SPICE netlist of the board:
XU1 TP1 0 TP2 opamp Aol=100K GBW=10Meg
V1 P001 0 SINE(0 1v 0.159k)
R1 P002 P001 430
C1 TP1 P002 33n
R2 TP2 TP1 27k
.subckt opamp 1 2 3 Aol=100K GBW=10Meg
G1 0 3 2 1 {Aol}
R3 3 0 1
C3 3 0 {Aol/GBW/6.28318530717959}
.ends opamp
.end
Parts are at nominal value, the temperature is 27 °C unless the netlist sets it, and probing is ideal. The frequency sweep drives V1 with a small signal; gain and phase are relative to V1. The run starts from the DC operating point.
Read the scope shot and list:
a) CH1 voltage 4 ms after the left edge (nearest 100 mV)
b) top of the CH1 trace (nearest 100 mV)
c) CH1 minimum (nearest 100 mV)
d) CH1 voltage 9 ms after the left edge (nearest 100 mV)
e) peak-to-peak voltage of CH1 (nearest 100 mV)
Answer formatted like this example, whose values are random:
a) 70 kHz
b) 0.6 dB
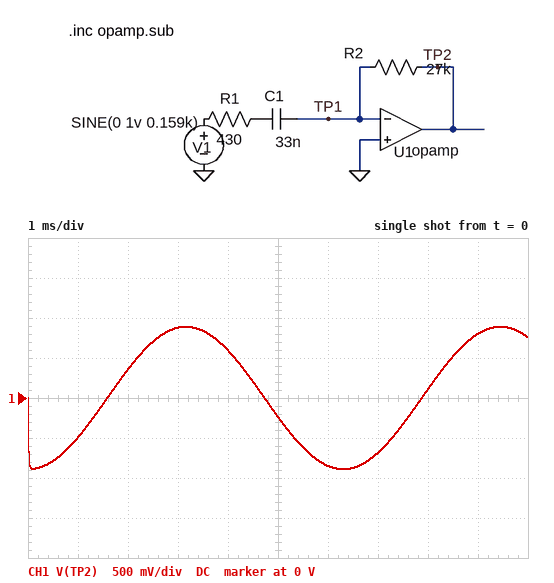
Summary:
a) 600 mV
b) 900 mV
c) -900 mV
d) 800 mV
e) 1.8 V
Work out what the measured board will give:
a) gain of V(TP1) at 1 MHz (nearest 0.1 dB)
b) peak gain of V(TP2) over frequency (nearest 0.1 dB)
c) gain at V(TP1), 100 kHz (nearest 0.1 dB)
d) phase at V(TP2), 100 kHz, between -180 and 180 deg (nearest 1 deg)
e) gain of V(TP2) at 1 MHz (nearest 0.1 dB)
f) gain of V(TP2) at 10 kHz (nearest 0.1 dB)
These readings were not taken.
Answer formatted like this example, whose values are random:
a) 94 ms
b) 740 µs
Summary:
a) -0.2 dB
b) 35.9 dB
c) -5.1 dB
d) 152 deg
e) 19.8 dB
f) 32.7 dB
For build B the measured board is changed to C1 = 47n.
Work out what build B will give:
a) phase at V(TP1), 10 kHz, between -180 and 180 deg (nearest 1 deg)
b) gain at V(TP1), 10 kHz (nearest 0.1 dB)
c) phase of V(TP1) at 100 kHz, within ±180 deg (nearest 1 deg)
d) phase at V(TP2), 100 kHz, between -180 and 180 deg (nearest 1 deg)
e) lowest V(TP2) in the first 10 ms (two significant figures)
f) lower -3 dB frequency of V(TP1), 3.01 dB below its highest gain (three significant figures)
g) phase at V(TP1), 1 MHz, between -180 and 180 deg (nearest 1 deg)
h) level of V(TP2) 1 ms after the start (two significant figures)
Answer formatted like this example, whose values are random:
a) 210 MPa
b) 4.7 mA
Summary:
a) 125 deg
b) -25.9 dB
c) 61 deg
d) 151 deg
e) -1.3 V
f) 149 kHz
g) 9 deg
h) -710 mV
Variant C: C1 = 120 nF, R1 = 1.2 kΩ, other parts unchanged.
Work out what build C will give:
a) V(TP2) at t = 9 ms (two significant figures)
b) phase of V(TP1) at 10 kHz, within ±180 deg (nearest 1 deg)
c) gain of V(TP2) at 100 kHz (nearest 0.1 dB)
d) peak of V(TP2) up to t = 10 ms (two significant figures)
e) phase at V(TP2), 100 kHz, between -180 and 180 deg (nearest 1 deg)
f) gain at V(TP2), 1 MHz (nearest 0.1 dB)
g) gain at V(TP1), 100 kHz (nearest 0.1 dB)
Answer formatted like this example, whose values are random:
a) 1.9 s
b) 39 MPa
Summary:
a) 2.7 V
b) 94 deg
c) 26.8 dB
d) 3.2 V
e) 167 deg
f) 18.9 dB
g) -13.2 dB
